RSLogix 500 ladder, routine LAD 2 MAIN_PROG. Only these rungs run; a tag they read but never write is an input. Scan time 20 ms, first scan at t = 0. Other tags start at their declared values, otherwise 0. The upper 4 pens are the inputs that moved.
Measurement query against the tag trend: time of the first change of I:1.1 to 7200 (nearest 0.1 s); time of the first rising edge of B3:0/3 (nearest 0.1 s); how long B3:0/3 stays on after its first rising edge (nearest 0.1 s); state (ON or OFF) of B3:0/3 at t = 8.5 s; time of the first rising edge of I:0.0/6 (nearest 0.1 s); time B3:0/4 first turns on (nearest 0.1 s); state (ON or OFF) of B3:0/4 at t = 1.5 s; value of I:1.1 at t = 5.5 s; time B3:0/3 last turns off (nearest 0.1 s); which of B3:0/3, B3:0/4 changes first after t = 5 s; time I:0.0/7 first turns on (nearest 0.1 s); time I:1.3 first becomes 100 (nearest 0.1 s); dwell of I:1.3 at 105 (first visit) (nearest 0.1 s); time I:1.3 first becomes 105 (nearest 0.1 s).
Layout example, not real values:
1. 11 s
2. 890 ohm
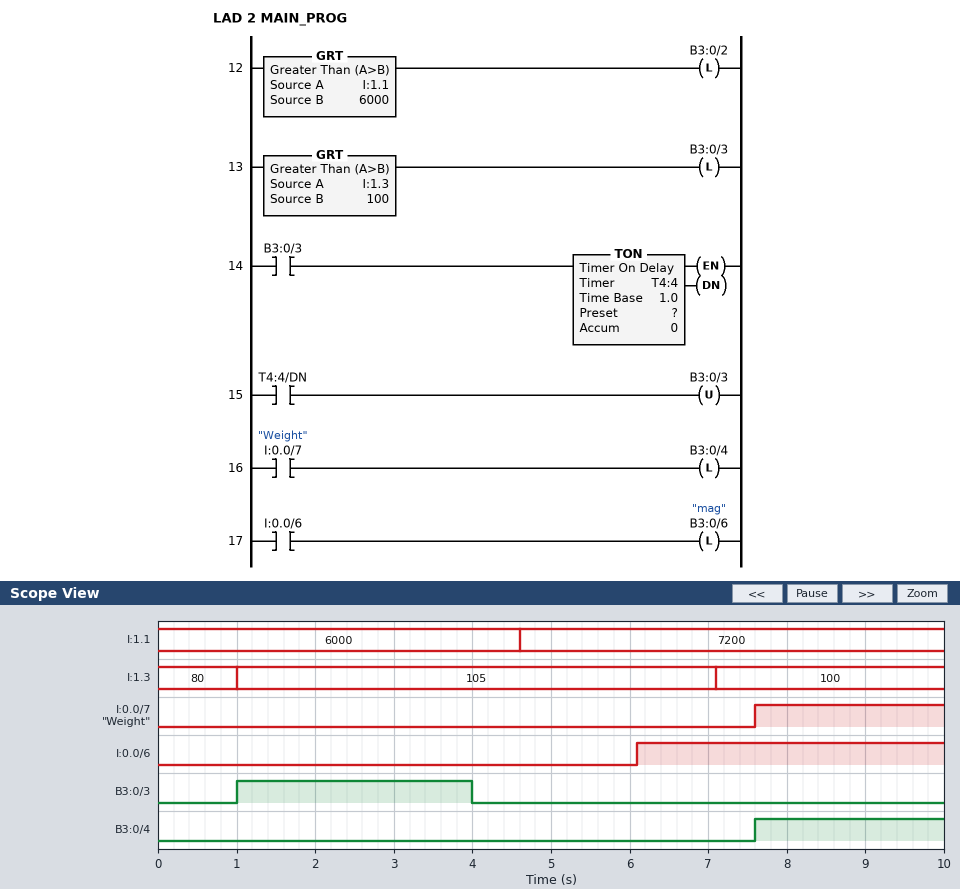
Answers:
1. 4.6 s
2. 1.0 s
3. 3.0 s
4. OFF
5. 6.1 s
6. 7.6 s
7. OFF
8. 7200
9. 4.0 s
10. B3:0/4
11. 7.6 s
12. 7.1 s
13. 6.1 s
14. 1.0 s
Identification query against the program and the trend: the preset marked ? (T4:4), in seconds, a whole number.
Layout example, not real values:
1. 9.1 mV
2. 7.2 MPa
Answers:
1. 3 s
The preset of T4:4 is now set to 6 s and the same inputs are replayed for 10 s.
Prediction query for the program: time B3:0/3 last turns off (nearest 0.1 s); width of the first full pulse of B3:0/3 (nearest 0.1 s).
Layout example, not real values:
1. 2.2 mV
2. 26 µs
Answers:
1. 7.0 s
2. 6.0 s
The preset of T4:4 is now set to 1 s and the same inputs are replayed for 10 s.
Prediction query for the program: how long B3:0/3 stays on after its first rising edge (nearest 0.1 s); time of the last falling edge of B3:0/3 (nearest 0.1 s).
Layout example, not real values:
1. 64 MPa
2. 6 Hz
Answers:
1. 1.0 s
2. 2.0 s
